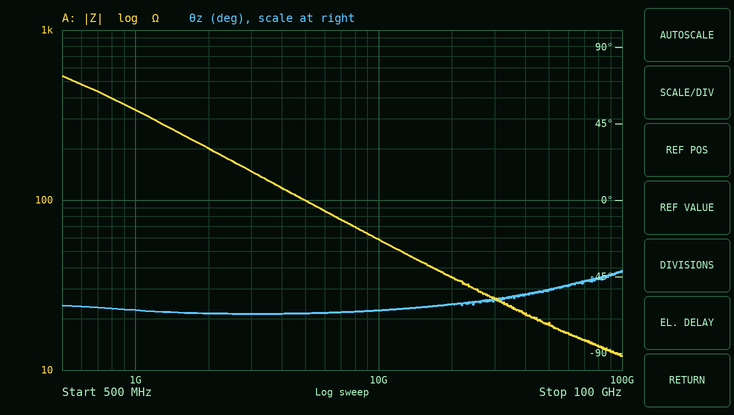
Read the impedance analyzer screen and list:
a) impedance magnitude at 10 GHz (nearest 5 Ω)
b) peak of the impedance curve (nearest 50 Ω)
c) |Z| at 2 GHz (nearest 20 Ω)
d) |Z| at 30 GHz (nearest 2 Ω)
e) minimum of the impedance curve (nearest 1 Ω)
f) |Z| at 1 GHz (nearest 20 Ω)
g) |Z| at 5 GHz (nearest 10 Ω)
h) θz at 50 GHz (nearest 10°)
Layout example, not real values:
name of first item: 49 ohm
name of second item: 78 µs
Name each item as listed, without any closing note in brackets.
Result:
impedance magnitude at 10 GHz: 60 Ω
peak of the impedance curve: 550 Ω
|Z| at 2 GHz: 200 Ω
|Z| at 30 GHz: 26 Ω
minimum of the impedance curve: 12 Ω
|Z| at 1 GHz: 340 Ω
|Z| at 5 GHz: 100 Ω
θz at 50 GHz: -50°
